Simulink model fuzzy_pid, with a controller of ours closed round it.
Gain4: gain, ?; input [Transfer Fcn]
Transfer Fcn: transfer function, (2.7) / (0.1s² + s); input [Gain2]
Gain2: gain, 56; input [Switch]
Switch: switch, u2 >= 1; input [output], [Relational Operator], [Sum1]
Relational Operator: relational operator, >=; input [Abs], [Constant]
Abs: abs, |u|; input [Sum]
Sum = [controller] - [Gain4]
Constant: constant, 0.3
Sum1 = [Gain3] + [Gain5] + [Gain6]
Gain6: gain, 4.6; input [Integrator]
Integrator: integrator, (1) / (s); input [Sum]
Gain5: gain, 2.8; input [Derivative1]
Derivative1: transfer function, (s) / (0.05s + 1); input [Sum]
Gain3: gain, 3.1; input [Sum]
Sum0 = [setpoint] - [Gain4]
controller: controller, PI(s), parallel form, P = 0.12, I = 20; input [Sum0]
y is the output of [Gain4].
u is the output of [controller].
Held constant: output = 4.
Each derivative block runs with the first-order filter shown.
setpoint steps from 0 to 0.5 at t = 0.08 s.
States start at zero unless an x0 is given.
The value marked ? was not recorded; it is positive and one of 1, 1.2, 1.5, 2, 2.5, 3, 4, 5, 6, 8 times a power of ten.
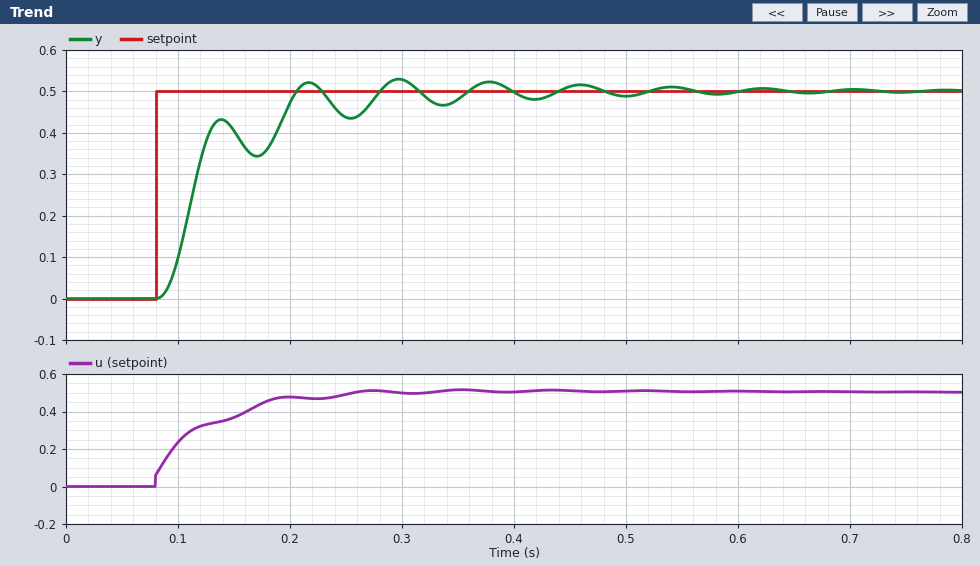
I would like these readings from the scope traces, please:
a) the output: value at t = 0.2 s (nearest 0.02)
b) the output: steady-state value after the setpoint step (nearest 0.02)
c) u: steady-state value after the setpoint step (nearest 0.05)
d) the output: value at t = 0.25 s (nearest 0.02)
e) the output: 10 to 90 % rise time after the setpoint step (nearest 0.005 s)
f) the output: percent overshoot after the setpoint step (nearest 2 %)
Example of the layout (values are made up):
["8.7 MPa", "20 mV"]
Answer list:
["0.48", "0.50", "0.50", "0.44", "0.100 s", "6 %"]
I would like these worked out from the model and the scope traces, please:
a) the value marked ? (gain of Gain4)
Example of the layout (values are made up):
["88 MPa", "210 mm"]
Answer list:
["0.06"]
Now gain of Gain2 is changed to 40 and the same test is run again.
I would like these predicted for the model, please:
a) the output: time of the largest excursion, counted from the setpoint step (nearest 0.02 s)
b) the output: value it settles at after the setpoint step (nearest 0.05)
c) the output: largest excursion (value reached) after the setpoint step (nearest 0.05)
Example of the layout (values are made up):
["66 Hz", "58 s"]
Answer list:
["0.16 s", "0.50", "0.55"]
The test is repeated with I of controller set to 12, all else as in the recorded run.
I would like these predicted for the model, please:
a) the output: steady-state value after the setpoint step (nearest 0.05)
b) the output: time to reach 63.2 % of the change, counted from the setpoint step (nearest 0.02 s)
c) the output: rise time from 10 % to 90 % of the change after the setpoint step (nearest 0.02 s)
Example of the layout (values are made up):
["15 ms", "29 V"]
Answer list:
["0.50", "0.10 s", "0.18 s"]
